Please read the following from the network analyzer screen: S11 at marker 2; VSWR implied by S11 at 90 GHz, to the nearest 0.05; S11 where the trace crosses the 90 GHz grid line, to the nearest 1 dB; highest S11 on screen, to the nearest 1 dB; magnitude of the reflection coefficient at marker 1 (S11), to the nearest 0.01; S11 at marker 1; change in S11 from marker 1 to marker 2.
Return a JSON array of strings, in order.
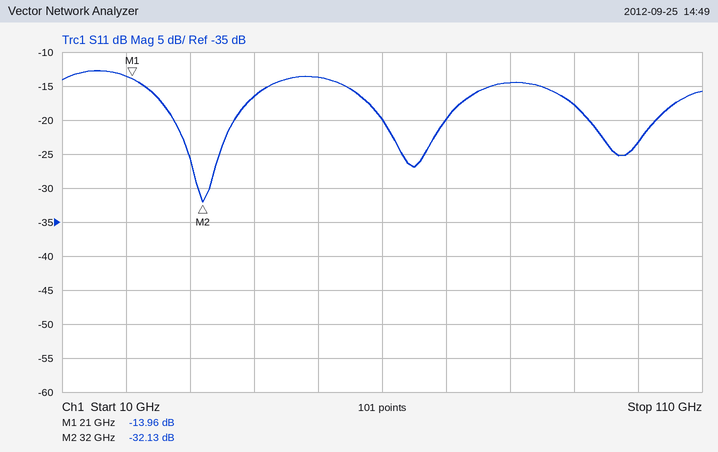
["-32.13 dB", "1.30", "-18 dB", "-13 dB", "0.20", "-13.96 dB", "-18.17 dB"]
